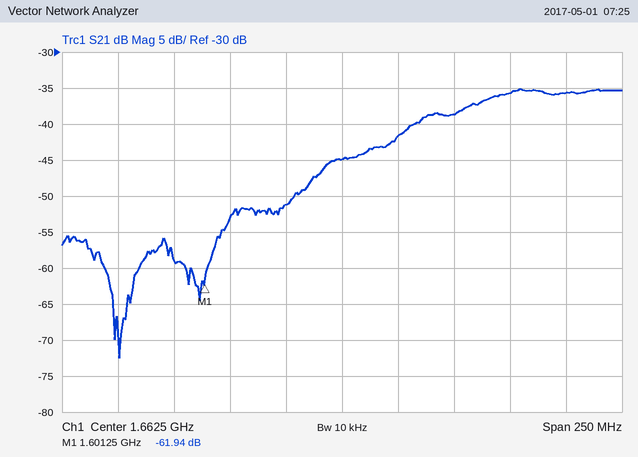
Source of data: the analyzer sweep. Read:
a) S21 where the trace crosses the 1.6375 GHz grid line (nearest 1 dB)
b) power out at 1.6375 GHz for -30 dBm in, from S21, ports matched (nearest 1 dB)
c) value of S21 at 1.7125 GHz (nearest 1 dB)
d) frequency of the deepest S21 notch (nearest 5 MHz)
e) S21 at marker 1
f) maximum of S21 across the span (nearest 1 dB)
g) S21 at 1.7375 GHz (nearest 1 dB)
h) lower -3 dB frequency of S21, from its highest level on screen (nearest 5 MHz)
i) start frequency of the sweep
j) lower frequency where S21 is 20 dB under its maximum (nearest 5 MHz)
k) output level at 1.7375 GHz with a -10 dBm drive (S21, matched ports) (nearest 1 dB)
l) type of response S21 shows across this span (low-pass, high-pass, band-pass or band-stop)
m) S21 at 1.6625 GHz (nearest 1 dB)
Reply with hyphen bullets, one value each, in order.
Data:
- -51 dB
- -81 dBm
- -39 dB
- 1.565 GHz
- -61.94 dB
- -35 dB
- -36 dB
- 1.715 GHz
- 1.5375 GHz
- 1.610 GHz
- -46 dBm
- high-pass
- -45 dB
